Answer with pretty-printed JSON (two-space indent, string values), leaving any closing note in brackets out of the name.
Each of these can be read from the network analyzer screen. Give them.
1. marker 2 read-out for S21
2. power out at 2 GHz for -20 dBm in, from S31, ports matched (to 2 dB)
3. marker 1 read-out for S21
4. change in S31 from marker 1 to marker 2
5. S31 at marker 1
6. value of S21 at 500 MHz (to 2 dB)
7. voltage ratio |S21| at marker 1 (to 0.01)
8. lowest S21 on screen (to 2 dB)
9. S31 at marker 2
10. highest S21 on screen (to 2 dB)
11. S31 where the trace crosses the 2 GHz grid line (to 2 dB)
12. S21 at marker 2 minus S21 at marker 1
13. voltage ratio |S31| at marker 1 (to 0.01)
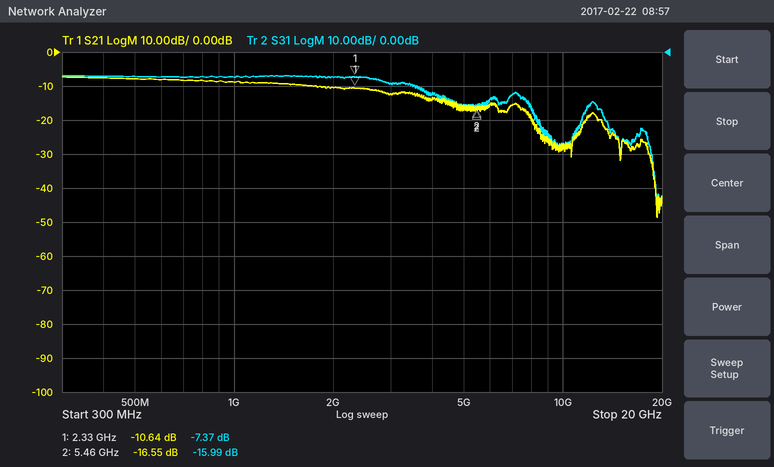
{
  "marker 2 read-out for S21": "-16.55 dB",
  "power out at 2 GHz for -20 dBm in, from S31, ports matched": "-28 dBm",
  "marker 1 read-out for S21": "-10.64 dB",
  "change in S31 from marker 1 to marker 2": "-8.62 dB",
  "S31 at marker 1": "-7.37 dB",
  "value of S21 at 500 MHz": "-8 dB",
  "voltage ratio |S21| at marker 1": "0.29",
  "lowest S21 on screen": "-48 dB",
  "S31 at marker 2": "-15.99 dB",
  "highest S21 on screen": "-8 dB",
  "S31 where the trace crosses the 2 GHz grid line": "-8 dB",
  "S21 at marker 2 minus S21 at marker 1": "-5.91 dB",
  "voltage ratio |S31| at marker 1": "0.43"
}
